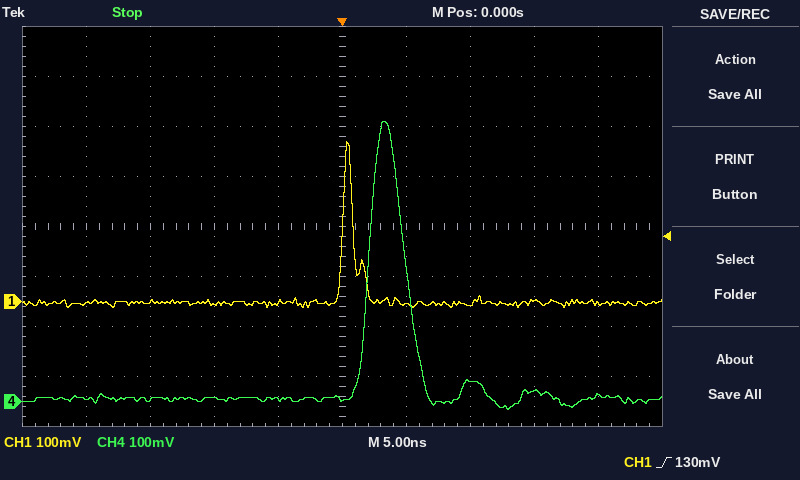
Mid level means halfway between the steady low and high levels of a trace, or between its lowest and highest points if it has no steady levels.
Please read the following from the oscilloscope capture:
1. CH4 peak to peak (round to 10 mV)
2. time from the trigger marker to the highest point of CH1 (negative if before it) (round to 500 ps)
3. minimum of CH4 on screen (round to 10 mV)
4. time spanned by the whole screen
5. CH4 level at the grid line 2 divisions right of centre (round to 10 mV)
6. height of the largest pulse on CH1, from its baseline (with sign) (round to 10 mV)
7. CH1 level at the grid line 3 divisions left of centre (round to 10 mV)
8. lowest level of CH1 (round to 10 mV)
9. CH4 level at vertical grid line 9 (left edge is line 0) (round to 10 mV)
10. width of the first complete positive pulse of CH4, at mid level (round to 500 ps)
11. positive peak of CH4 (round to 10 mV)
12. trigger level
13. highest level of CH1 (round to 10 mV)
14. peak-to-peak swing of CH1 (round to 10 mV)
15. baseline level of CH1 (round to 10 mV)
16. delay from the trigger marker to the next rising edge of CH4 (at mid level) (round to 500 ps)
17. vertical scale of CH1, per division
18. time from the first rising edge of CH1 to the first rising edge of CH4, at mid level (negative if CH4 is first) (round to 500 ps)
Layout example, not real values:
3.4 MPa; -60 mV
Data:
580 mV; +500 ps; -20 mV; 50 ns; 40 mV; +320 mV; 0 mV; -10 mV; 10 mV; 3.0 ns; 560 mV; 130 mV; 320 mV; 330 mV; 0 mV; 2.0 ns; 100 mV; +2.0 ns
